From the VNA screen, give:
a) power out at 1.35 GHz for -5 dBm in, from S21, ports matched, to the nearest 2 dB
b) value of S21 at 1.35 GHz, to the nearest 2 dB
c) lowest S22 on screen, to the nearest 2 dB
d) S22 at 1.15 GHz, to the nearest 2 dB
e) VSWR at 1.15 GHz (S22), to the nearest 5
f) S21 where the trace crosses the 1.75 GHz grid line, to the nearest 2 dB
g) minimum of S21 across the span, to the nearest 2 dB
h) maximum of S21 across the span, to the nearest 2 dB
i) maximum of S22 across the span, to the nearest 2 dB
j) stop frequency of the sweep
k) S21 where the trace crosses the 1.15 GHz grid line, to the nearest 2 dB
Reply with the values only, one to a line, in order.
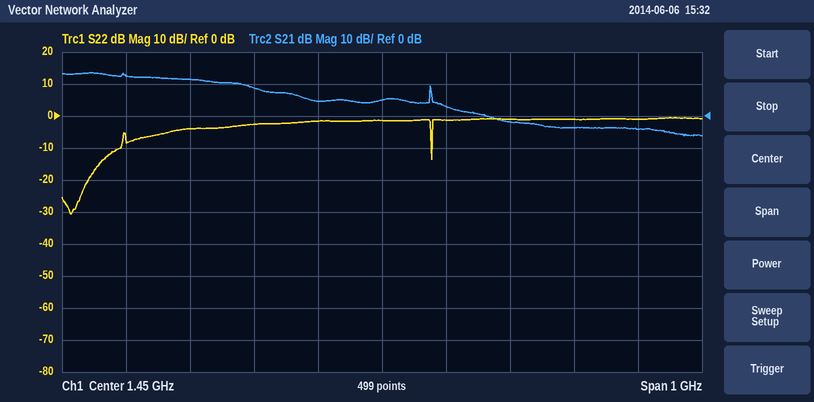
0 dBm
4 dB
-30 dB
-4 dB
5
-4 dB
-6 dB
14 dB
0 dB
1.95 GHz
12 dB
